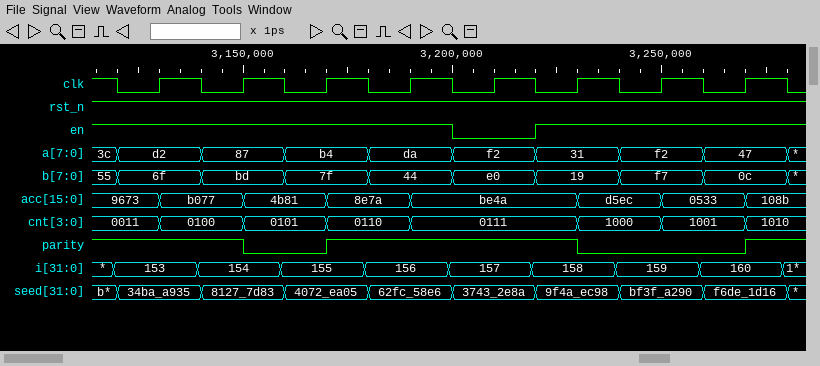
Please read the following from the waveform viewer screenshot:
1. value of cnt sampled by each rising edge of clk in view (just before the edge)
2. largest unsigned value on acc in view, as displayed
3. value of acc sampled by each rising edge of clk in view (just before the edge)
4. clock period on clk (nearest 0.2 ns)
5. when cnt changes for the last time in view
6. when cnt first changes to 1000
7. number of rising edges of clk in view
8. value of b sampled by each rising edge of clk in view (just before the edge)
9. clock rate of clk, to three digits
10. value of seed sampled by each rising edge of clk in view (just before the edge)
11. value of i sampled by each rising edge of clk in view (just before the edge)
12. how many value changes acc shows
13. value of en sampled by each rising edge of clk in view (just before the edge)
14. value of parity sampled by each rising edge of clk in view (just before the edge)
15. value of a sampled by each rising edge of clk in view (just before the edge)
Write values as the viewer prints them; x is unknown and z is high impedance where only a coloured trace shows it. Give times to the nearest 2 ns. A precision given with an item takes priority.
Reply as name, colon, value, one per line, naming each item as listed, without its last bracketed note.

value of cnt sampled by each rising edge of clk in view: 0011, 0100, 0101, 0110, 0111, 0111, 1000, 1001
largest unsigned value on acc in view, as displayed: d5ec
value of acc sampled by each rising edge of clk in view: 9673, b077, 4b81, 8e7a, be4a, be4a, d5ec, 0533
clock period on clk: 20 ns
when cnt changes for the last time in view: 3270 ns
when cnt first changes to 1000: 3230 ns
number of rising edges of clk in view: 8
value of b sampled by each rising edge of clk in view: 6f, bd, 7f, 44, e0, 19, f7, 0c
clock rate of clk, to three digits: 50.0 MHz
value of seed sampled by each rising edge of clk in view: 34ba_a935, 8127_7d83, 4072_ea05, 62fc_58e6, 3743_2e8a, 9f4a_ec98, bf3f_a290, f6de_1d16
value of i sampled by each rising edge of clk in view: 153, 154, 155, 156, 157, 158, 159, 160
how many value changes acc shows: 7
value of en sampled by each rising edge of clk in view: 1 1 1 1 0 1 1 1
value of parity sampled by each rising edge of clk in view: 1 1 0 1 1 1 0 0
value of a sampled by each rising edge of clk in view: d2, 87, b4, da, f2, 31, f2, 47
